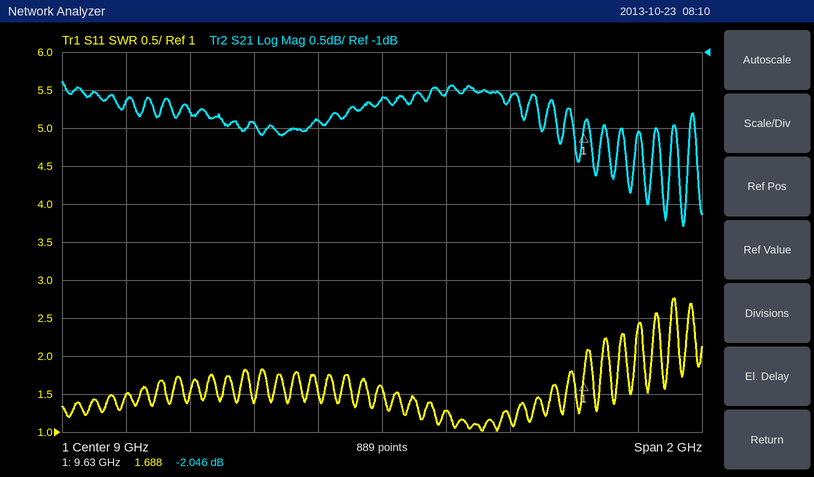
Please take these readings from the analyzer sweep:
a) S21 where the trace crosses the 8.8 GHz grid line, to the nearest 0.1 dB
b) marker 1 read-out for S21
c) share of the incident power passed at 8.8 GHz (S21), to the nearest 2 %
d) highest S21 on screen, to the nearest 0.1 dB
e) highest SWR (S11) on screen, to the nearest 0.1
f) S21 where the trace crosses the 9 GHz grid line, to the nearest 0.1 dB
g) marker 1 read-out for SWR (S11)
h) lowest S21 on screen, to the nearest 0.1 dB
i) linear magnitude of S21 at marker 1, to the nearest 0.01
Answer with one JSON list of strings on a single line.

["-1.9 dB", "-2.046 dB", "64 %", "-1.4 dB", "2.8", "-1.6 dB", "1.688", "-3.3 dB", "0.79"]
